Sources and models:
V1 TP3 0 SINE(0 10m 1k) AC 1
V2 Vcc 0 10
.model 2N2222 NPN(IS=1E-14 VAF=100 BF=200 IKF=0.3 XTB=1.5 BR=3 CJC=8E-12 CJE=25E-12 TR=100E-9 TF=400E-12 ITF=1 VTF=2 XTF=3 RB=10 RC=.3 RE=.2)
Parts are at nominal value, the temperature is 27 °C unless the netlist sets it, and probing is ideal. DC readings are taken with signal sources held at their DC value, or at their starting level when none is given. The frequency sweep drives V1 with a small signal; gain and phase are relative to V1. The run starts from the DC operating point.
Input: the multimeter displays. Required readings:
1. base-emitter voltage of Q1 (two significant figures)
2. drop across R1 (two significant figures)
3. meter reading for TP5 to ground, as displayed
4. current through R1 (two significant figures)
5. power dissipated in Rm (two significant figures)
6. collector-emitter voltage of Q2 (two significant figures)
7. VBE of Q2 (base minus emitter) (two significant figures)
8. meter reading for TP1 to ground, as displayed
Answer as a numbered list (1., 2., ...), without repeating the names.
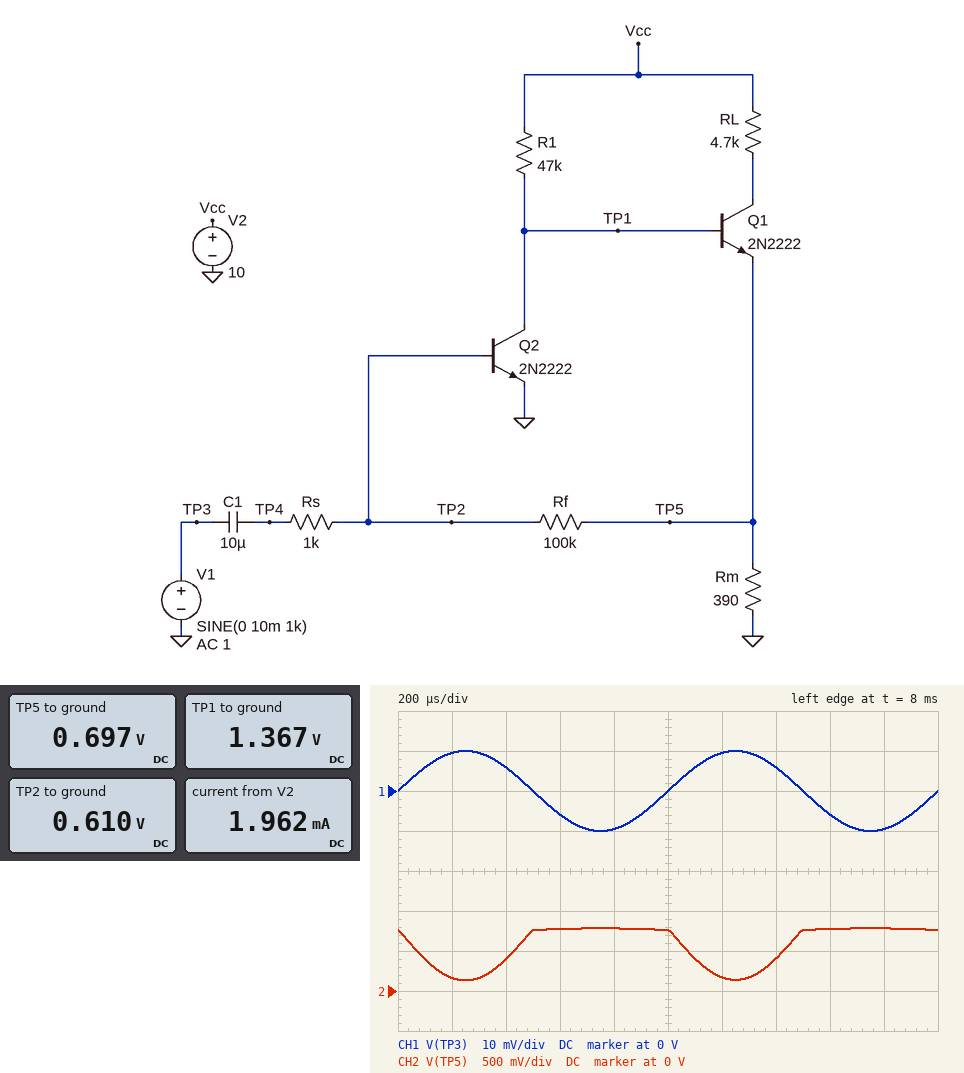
1. 670 mV
2. 8.6 V
3. 0.697 V
4. 180 µA
5. 1.2 mW
6. 1.4 V
7. 610 mV
8. 1.367 V
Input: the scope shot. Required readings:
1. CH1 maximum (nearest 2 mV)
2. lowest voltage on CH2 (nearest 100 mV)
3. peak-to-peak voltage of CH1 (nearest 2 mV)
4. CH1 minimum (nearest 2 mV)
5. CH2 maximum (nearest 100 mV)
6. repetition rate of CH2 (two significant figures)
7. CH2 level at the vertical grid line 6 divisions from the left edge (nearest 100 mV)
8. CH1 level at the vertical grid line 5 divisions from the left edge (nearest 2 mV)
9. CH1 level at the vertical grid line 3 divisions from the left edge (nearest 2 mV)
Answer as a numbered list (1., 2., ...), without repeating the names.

1. 10 mV
2. 100 mV
3. 20 mV
4. -10 mV
5. 800 mV
6. 1.0 kHz
7. 200 mV
8. 0 V
9. -6 mV
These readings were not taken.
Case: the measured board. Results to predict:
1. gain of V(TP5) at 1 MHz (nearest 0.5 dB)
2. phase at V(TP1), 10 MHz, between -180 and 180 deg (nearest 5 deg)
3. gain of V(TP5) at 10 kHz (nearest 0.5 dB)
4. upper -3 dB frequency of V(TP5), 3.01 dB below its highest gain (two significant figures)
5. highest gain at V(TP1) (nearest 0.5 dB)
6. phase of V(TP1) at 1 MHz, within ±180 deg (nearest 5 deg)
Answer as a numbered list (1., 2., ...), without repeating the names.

1. 16.5 dB
2. 80 deg
3. 36.0 dB
4. 110 kHz
5. 36.5 dB
6. 95 deg
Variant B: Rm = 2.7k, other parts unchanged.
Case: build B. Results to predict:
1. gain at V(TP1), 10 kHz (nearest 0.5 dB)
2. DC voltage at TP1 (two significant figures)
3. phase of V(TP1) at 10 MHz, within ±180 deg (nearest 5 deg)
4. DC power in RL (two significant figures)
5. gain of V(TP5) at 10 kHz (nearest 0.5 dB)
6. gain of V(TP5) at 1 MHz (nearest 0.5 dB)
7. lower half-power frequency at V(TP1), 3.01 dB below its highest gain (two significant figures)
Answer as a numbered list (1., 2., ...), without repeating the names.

1. 37.5 dB
2. 1.3 V
3. 70 deg
4. 320 µW
5. 37.0 dB
6. 24.0 dB
7. 12 Hz
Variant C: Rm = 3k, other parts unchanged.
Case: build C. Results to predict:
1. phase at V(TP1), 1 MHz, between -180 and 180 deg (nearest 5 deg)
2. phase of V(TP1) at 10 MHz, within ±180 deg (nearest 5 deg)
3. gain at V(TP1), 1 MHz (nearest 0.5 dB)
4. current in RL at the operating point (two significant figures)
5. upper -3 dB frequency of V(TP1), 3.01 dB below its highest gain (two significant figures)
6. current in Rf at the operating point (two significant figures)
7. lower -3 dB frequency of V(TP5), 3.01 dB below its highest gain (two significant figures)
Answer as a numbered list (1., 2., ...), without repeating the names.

1. 100 deg
2. 70 deg
3. 24.5 dB
4. 230 µA
5. 230 kHz
6. 910 nA
7. 12 Hz
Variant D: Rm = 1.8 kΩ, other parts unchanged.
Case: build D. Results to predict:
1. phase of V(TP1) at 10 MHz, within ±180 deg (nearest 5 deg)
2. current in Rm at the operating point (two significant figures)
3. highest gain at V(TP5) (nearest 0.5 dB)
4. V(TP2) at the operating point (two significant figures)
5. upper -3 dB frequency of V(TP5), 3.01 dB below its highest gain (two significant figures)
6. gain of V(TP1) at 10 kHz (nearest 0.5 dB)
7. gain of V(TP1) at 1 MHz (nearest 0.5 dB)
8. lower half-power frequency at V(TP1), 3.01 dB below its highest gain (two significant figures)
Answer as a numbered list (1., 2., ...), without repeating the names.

1. 70 deg
2. 390 µA
3. 37.0 dB
4. 610 mV
5. 220 kHz
6. 37.5 dB
7. 24.0 dB
8. 12 Hz
